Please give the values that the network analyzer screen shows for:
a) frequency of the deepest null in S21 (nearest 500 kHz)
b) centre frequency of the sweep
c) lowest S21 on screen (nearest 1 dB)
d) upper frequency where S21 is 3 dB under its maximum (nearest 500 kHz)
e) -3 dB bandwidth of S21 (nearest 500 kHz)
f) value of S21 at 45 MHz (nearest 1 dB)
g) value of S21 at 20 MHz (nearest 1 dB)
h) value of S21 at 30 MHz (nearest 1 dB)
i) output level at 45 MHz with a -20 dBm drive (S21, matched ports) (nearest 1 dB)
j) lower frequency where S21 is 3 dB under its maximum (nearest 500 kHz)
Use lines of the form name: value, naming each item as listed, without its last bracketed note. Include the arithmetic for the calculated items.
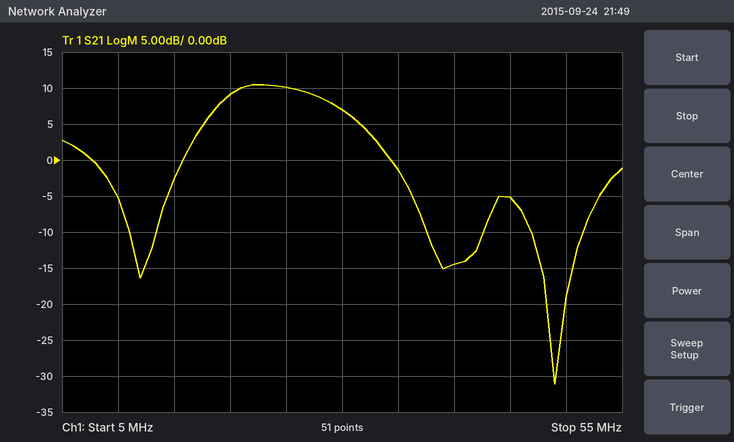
frequency of the deepest null in S21: 49.0 MHz
centre frequency of the sweep: 30 MHz
lowest S21 on screen: -31 dB
upper frequency where S21 is 3 dB under its maximum: 29.5 MHz
-3 dB bandwidth of S21: 29.5 MHz − 19.0 MHz = 10.5 MHz
value of S21 at 45 MHz: -5 dB
value of S21 at 20 MHz: 9 dB
value of S21 at 30 MHz: 7 dB
output level at 45 MHz with a -20 dBm drive (S21, matched ports): -20 dBm + (-5 dB) = -25 dBm
lower frequency where S21 is 3 dB under its maximum: 19.0 MHz
